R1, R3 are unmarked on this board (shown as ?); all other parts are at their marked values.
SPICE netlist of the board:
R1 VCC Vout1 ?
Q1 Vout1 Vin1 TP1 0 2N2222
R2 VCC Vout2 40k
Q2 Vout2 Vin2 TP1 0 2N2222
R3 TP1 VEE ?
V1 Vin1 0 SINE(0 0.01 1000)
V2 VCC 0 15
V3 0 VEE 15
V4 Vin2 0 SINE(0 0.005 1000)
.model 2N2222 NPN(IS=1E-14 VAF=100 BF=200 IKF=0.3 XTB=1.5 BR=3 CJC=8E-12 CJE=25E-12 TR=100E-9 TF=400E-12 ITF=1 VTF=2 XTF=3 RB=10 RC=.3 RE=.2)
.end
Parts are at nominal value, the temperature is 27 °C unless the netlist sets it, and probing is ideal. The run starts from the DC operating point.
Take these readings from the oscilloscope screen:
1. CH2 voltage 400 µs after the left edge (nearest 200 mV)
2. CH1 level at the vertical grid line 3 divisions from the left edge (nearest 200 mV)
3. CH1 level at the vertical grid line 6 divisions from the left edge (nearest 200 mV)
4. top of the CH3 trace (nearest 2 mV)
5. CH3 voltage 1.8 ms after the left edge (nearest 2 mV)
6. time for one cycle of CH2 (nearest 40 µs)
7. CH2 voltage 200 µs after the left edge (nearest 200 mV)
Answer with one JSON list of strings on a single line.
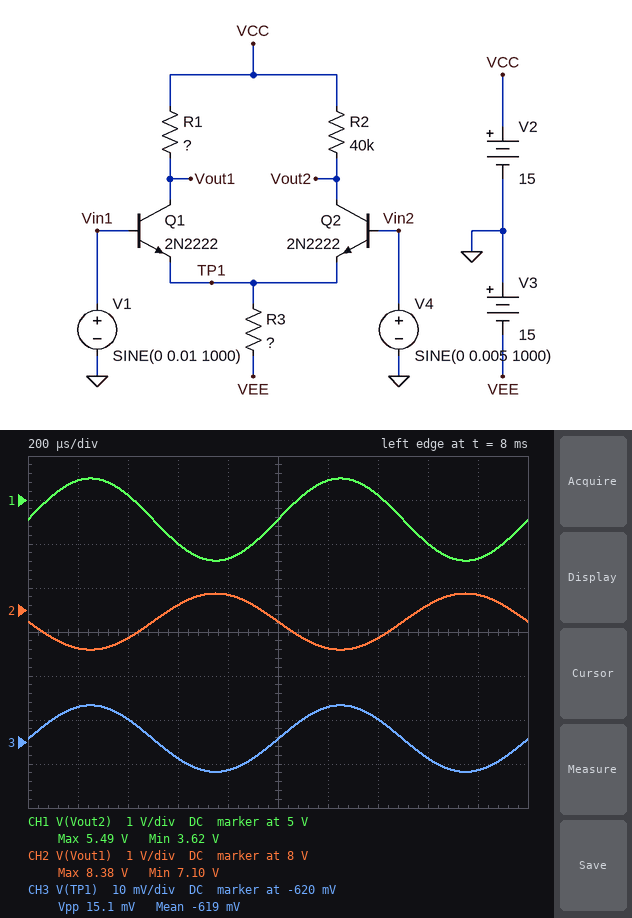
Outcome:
["7.4 V", "4.0 V", "5.4 V", "-612 mV", "-626 mV", "1.00 ms", "7.2 V"]
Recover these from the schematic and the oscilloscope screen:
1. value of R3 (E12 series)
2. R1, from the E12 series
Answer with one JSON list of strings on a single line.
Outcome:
["27 kΩ", "27 kΩ"]
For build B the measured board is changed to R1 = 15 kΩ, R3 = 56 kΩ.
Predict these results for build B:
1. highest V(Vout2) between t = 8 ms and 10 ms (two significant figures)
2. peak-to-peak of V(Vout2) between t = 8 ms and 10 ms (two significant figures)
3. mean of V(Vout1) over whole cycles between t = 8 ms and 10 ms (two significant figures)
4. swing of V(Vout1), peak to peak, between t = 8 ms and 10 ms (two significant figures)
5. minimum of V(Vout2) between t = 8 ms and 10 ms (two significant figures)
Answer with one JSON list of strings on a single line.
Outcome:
["10 V", "950 mV", "13 V", "360 mV", "9.5 V"]
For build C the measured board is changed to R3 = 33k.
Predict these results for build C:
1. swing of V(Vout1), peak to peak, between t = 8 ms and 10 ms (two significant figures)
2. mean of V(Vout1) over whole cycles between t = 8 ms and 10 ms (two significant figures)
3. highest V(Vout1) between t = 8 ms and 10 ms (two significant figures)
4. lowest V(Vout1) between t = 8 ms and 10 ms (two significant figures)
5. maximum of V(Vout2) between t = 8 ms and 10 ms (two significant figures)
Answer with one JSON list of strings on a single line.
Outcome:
["1.1 V", "9.1 V", "9.6 V", "8.5 V", "7.2 V"]
